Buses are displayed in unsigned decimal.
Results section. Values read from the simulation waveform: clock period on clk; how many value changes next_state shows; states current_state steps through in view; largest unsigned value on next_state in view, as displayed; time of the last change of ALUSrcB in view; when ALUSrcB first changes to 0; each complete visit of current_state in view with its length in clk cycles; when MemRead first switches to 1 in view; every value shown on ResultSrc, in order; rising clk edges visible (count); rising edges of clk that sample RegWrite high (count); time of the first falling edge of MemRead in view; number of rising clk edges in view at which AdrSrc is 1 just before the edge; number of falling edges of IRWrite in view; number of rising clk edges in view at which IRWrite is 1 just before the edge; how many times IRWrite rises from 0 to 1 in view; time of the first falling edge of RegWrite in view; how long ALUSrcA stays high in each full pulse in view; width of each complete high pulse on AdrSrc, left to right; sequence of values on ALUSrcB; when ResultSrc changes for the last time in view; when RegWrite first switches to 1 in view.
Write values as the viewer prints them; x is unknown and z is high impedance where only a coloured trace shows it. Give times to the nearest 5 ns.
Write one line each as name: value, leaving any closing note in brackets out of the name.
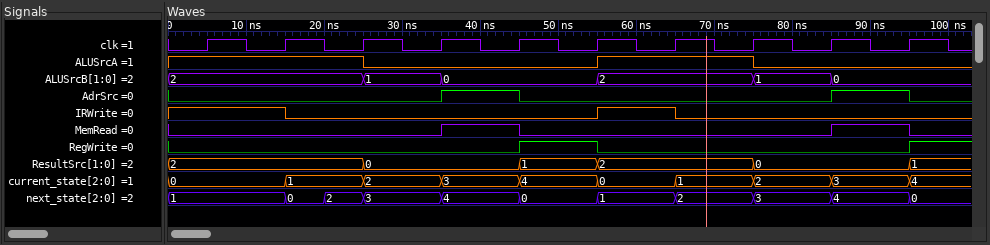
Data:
clock period on clk: 10 ns
how many value changes next_state shows: 10
states current_state steps through in view: 0, 1, 2, 3, 4, 0, 1, 2, 3, 4
largest unsigned value on next_state in view, as displayed: 4
time of the last change of ALUSrcB in view: 85 ns
when ALUSrcB first changes to 0: 35 ns
each complete visit of current_state in view with its length in clk cycles: 1: 1, 2: 1, 3: 1, 4: 1, 0: 1, 1: 1, 2: 1, 3: 1
when MemRead first switches to 1 in view: 35 ns
every value shown on ResultSrc, in order: 2, 0, 1, 2, 0, 1
rising clk edges visible: 10
rising edges of clk that sample RegWrite high: 1
time of the first falling edge of MemRead in view: 45 ns
number of rising clk edges in view at which AdrSrc is 1 just before the edge: 2
number of falling edges of IRWrite in view: 2
number of rising clk edges in view at which IRWrite is 1 just before the edge: 3
how many times IRWrite rises from 0 to 1 in view: 1
time of the first falling edge of RegWrite in view: 55 ns
how long ALUSrcA stays high in each full pulse in view: 20 ns
width of each complete high pulse on AdrSrc, left to right: 10 ns, 10 ns
sequence of values on ALUSrcB: 2, 1, 0, 2, 1, 0
when ResultSrc changes for the last time in view: 95 ns
when RegWrite first switches to 1 in view: 45 ns
